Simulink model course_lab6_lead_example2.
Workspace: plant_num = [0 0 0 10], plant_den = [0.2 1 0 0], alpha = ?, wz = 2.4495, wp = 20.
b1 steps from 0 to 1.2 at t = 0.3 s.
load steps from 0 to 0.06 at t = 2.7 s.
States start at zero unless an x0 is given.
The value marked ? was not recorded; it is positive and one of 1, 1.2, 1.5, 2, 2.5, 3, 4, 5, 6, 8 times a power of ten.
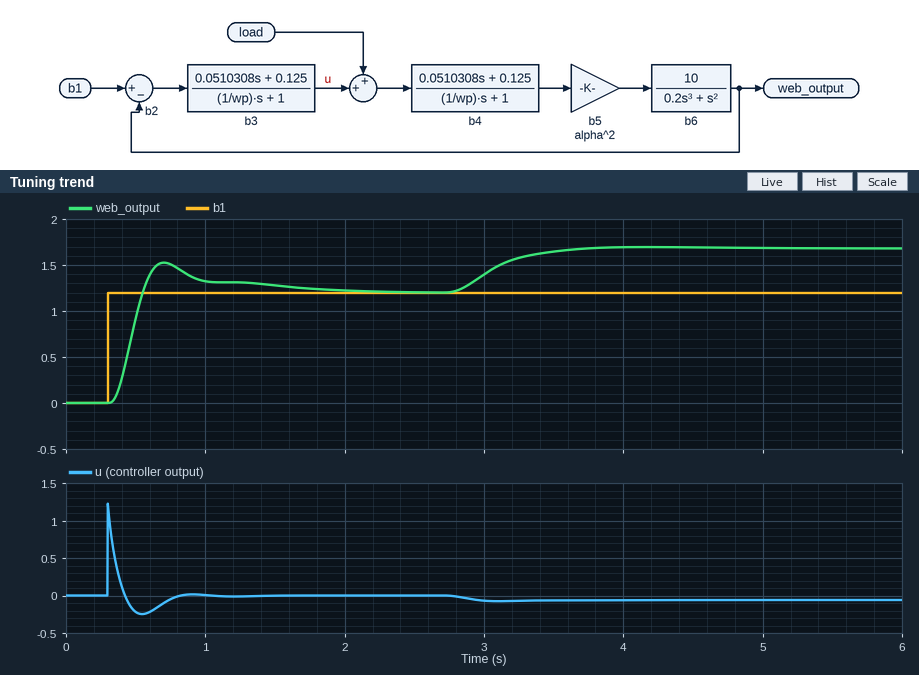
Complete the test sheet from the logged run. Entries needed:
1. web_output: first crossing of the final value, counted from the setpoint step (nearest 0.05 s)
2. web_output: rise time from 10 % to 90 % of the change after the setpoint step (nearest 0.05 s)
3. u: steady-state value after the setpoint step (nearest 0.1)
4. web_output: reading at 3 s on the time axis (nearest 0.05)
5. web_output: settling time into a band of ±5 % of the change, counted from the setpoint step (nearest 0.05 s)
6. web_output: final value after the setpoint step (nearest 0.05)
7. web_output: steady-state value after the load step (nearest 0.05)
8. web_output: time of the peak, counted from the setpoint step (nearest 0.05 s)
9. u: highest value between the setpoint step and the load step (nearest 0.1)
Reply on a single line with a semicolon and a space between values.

0.25 s; 0.15 s; 0.0; 1.40; 1.30 s; 1.20; 1.70; 0.40 s; 1.2
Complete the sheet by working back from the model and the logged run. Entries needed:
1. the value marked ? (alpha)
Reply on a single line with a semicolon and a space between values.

8
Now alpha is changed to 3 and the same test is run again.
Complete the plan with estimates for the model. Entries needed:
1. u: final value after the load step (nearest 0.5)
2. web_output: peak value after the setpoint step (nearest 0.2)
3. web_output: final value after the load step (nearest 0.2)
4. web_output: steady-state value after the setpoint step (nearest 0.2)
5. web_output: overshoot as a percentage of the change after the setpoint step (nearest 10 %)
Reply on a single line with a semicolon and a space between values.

0.0; 1.6; 1.4; 1.2; 30 %
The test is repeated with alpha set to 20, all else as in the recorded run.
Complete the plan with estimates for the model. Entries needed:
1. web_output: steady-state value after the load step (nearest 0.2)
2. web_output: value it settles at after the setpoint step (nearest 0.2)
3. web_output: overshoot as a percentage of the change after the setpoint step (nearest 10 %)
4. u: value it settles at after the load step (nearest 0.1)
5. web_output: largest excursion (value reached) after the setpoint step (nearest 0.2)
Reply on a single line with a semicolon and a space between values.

2.4; 1.2; 30 %; -0.1; 1.6
